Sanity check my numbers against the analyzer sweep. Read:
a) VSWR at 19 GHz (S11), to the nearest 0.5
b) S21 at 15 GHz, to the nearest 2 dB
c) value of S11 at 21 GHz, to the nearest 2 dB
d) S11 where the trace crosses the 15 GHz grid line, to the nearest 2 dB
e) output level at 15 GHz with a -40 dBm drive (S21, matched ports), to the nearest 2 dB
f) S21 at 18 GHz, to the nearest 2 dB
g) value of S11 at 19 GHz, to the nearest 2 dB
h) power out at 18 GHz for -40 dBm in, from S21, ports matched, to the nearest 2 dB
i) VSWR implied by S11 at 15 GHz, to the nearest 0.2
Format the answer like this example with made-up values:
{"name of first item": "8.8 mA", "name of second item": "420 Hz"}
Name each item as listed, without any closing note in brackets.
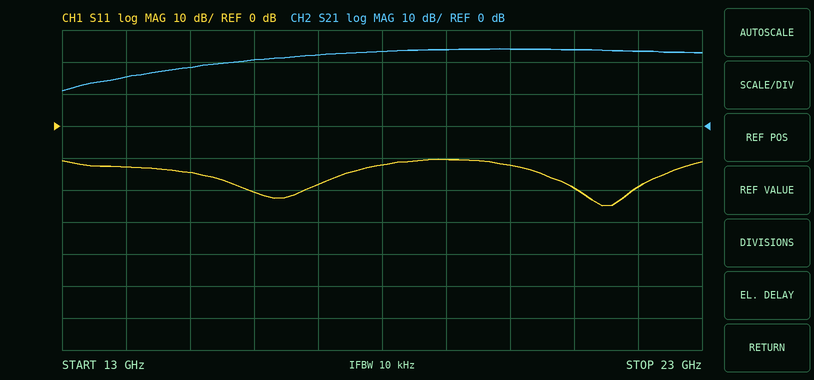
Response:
{"VSWR at 19 GHz (S11), to the nearest 0.5": "2.0", "S21 at 15 GHz, to the nearest 2 dB": "18 dB", "value of S11 at 21 GHz, to the nearest 2 dB": "-20 dB", "S11 where the trace crosses the 15 GHz grid line, to the nearest 2 dB": "-14 dB", "output level at 15 GHz with a -40 dBm drive (S21, matched ports), to the nearest 2 dB": "-22 dBm", "S21 at 18 GHz, to the nearest 2 dB": "24 dB", "value of S11 at 19 GHz, to the nearest 2 dB": "-10 dB", "power out at 18 GHz for -40 dBm in, from S21, ports matched, to the nearest 2 dB": "-16 dBm", "VSWR implied by S11 at 15 GHz, to the nearest 0.2": "1.4"}
